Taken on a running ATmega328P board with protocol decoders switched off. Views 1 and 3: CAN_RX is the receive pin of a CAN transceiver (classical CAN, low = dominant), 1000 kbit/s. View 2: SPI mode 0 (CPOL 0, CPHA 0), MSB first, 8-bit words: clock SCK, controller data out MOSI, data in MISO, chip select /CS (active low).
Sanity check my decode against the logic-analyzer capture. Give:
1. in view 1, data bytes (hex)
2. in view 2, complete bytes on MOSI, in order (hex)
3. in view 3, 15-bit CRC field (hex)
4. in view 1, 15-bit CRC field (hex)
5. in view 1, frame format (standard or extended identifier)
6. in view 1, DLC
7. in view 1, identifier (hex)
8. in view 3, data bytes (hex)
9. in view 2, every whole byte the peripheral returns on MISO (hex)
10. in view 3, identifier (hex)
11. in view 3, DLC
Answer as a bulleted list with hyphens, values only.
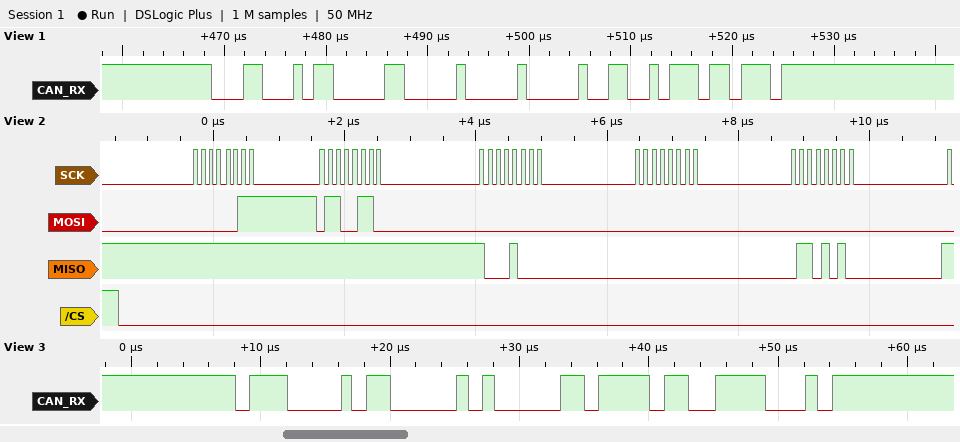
- 00 00
- 03 66 00 00 00
- 0x7678
- 0x65DB
- standard
- 2
- 0x18B
- 05
- FF FF 88 00 6A
- 0x70B
- 1
